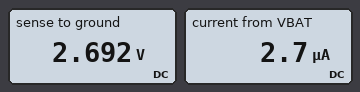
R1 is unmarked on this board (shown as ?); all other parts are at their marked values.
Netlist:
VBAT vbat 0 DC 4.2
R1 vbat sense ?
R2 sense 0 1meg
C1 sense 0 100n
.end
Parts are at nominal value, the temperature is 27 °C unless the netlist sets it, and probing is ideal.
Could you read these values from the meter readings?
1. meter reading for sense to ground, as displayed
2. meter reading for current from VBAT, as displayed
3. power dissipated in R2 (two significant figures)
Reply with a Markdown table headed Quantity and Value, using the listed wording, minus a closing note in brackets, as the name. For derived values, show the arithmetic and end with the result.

| Quantity | Value |
|---|---|
| meter reading for sense to ground, as displayed | 2.692 V |
| meter reading for current from VBAT, as displayed | 2.7 µA |
| power dissipated in R2 | (2.692 V)^2 / 1 MΩ = 7.2 µW |
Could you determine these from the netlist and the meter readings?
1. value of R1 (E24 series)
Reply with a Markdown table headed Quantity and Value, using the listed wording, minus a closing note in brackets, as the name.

| Quantity | Value |
|---|---|
| value of R1 | 560 kΩ |
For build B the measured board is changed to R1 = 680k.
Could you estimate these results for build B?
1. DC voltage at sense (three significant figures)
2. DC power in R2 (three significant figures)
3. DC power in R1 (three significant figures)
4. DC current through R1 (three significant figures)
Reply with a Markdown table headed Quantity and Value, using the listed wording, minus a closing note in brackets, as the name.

| Quantity | Value |
|---|---|
| DC voltage at sense | 2.50 V |
| DC power in R2 | 6.25 µW |
| DC power in R1 | 4.25 µW |
| DC current through R1 | 2.50 µA |
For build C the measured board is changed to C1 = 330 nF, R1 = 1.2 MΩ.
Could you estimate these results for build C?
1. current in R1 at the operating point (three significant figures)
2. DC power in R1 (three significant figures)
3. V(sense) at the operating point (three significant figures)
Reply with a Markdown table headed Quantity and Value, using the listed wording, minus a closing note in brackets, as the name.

| Quantity | Value |
|---|---|
| current in R1 at the operating point | 1.91 µA |
| DC power in R1 | 4.37 µW |
| V(sense) at the operating point | 1.91 V |
